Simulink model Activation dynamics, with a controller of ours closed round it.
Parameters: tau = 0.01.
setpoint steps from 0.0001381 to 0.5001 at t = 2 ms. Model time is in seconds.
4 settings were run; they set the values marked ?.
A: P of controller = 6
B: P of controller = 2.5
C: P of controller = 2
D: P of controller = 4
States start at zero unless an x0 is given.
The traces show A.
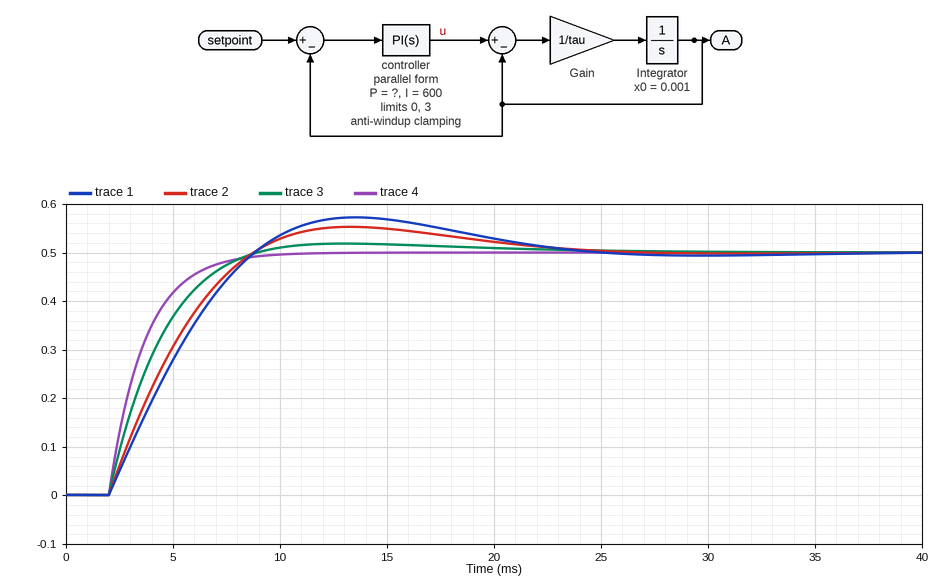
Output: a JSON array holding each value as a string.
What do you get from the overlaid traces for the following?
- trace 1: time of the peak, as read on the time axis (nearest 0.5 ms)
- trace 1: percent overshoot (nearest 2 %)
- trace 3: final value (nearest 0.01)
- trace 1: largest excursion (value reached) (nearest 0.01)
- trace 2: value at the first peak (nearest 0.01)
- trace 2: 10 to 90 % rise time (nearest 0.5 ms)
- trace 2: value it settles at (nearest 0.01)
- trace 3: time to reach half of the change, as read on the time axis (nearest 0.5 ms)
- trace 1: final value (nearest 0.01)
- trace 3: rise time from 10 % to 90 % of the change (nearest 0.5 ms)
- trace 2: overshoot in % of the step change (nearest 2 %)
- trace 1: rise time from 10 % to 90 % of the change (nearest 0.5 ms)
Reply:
["13.5 ms", "14 %", "0.50", "0.57", "0.55", "5.0 ms", "0.50", "3.5 ms", "0.50", "4.5 ms", "10 %", "5.0 ms"]
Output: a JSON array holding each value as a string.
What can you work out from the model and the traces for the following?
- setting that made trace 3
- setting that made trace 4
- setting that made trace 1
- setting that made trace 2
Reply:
["D", "A", "C", "B"]
